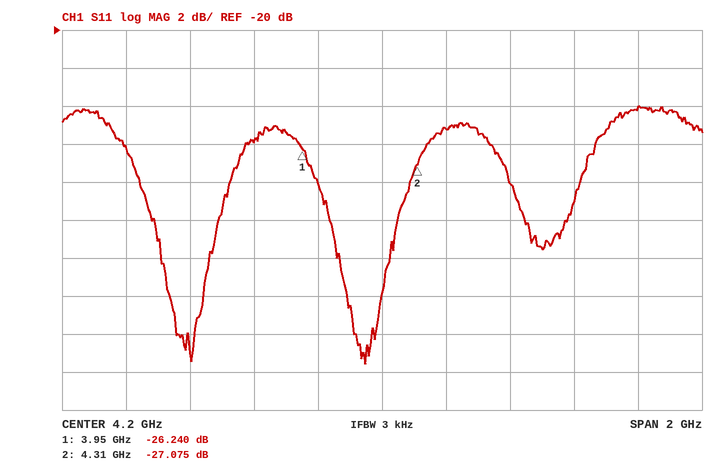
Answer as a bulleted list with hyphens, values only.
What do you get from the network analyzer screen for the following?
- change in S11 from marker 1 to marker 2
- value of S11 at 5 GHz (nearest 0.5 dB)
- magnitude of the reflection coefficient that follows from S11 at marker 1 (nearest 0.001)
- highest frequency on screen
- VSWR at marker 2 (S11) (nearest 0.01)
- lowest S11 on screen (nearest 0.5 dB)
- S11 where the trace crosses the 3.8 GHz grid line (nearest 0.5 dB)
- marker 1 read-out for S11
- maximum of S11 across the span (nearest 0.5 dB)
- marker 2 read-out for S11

- -0.835 dB
- -24.0 dB
- 0.049
- 5.2 GHz
- 1.09
- -37.5 dB
- -26.0 dB
- -26.240 dB
- -24.0 dB
- -27.075 dB
